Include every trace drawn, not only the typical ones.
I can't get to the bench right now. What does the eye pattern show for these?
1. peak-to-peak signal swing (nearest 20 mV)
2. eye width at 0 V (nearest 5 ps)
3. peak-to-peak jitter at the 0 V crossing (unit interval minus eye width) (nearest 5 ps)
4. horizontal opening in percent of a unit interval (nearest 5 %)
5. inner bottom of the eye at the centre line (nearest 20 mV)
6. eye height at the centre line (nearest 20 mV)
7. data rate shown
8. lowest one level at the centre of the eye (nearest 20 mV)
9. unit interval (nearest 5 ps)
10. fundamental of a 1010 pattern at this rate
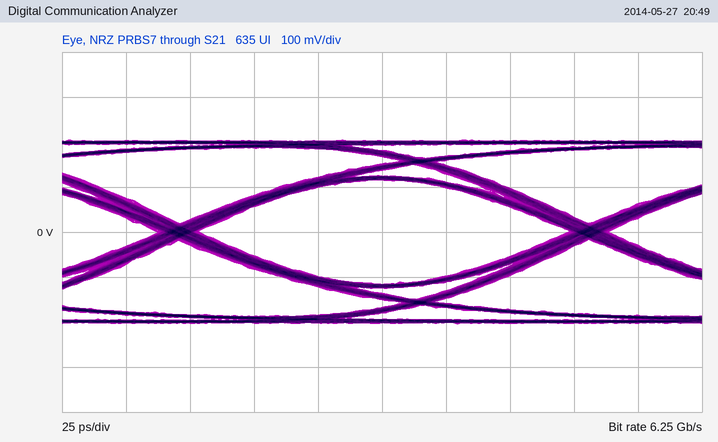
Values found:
400 mV
145 ps
15 ps
90 %
-120 mV
240 mV
6.25 Gb/s
120 mV
160 ps
3.125 GHz
